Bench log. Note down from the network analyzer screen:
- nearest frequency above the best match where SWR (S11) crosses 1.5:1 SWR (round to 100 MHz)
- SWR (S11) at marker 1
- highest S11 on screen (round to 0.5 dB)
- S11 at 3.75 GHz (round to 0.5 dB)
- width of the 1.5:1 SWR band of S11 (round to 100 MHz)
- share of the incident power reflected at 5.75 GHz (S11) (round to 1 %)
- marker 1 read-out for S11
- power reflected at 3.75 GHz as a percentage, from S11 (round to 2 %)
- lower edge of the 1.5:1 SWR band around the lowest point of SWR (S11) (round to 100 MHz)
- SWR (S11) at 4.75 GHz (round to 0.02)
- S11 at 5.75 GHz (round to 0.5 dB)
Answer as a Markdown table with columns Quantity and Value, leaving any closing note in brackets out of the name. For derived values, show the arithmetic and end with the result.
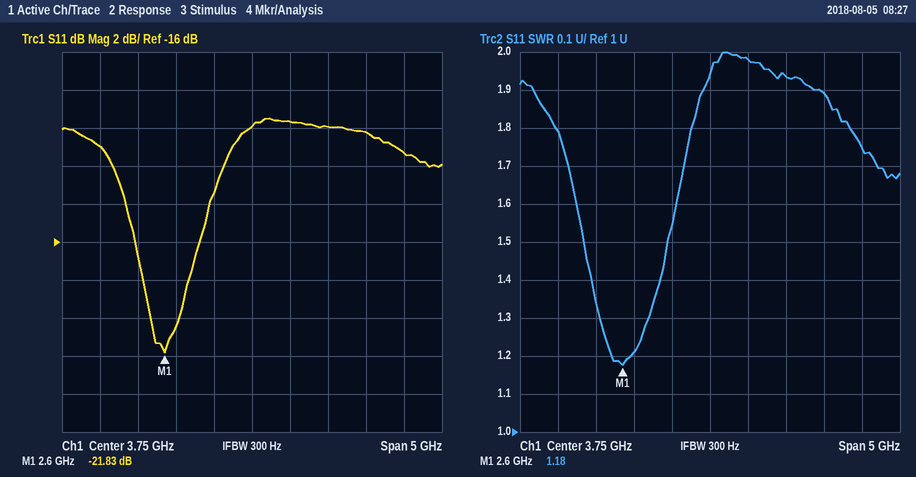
| Quantity | Value |
|---|---|
| nearest frequency above the best match where SWR (S11) crosses 1.5:1 SWR | 3.2 GHz |
| SWR (S11) at marker 1 | 1.18 |
| highest S11 on screen | -9.5 dB |
| S11 at 3.75 GHz | -10.0 dB |
| width of the 1.5:1 SWR band of S11 | 3.2 GHz − 2.1 GHz = 1.1 GHz |
| share of the incident power reflected at 5.75 GHz (S11) | 10^(-11.5/10) ≈ 7 % |
| marker 1 read-out for S11 | -21.83 dB |
| power reflected at 3.75 GHz as a percentage, from S11 | 10^(-10/10) ≈ 10 % |
| lower edge of the 1.5:1 SWR band around the lowest point of SWR (S11) | 2.1 GHz |
| SWR (S11) at 4.75 GHz | 1.94 |
| S11 at 5.75 GHz | -11.5 dB |
